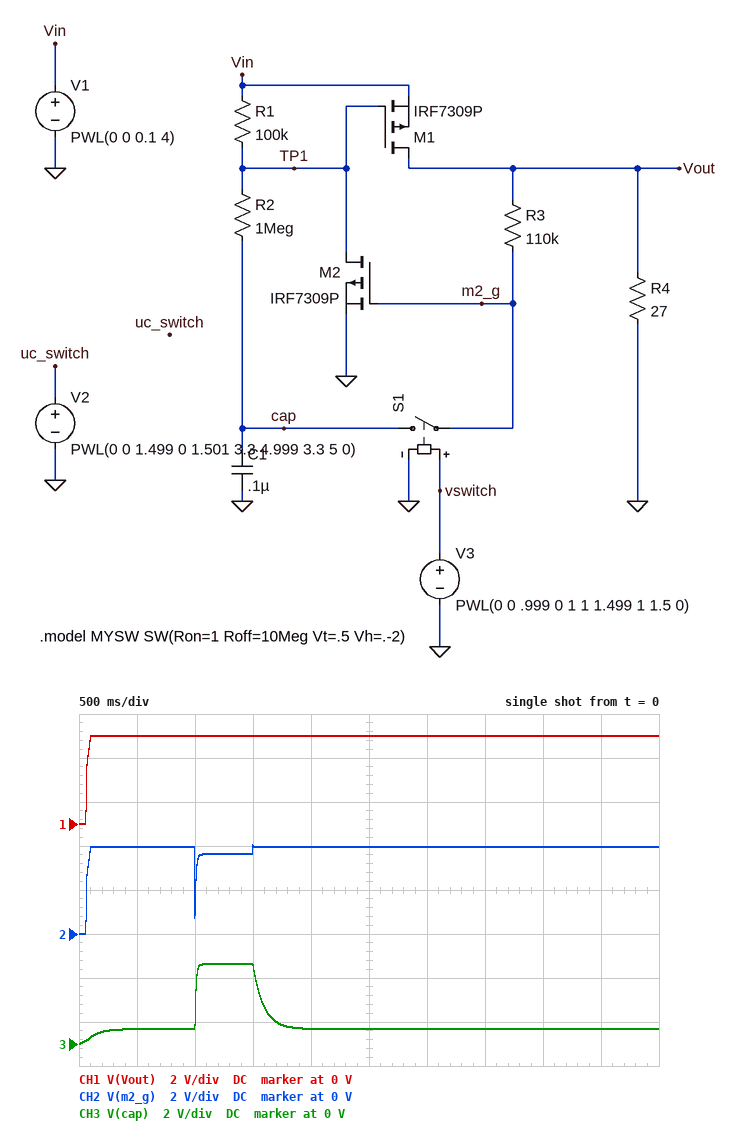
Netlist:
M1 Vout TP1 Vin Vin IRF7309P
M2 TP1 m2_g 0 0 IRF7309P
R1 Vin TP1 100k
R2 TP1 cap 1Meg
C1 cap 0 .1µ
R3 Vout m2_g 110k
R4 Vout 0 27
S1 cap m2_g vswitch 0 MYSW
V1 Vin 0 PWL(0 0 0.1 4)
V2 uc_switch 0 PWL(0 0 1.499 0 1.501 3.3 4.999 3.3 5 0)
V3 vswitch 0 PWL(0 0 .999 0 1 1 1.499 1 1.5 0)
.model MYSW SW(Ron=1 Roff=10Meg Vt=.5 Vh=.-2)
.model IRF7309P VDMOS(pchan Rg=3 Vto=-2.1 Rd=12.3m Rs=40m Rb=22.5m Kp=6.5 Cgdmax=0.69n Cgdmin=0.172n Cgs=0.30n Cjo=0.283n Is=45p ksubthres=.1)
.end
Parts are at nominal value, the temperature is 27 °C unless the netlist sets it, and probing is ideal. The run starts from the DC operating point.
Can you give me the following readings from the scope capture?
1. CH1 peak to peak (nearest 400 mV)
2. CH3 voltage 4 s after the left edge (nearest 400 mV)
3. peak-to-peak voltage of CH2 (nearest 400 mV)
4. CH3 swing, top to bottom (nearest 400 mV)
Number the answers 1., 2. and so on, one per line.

1. 4.0 V
2. 800 mV
3. 4.0 V
4. 3.6 V
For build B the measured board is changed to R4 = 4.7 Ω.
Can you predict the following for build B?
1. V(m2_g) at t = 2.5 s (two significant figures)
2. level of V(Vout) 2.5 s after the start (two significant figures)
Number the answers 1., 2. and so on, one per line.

1. 3.8 V
2. 3.9 V
